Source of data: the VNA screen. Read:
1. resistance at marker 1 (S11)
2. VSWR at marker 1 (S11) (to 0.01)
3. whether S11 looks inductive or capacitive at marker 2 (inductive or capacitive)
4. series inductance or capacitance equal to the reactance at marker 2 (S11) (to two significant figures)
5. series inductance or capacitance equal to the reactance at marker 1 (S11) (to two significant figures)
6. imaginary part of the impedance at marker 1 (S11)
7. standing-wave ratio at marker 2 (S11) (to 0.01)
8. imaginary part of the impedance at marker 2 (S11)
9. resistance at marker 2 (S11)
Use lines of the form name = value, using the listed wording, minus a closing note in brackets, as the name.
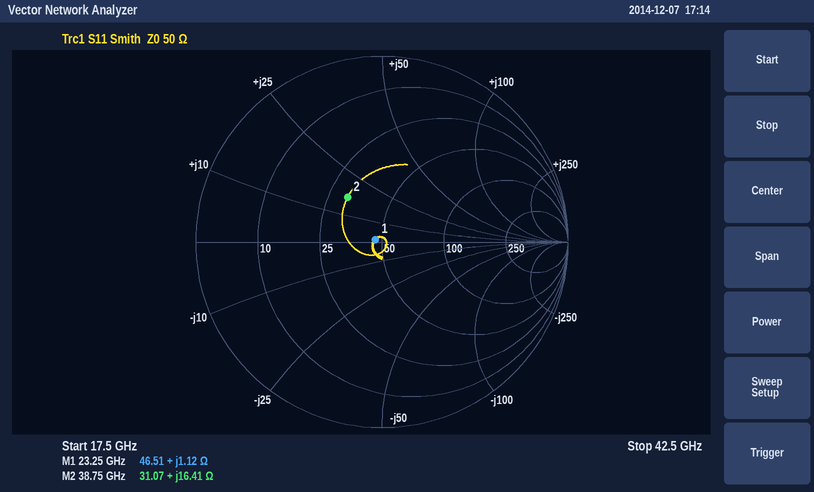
resistance at marker 1 = 46.51 Ω
VSWR at marker 1 (S11) = 1.08
whether S11 looks inductive or capacitive at marker 2 = inductive
series inductance or capacitance equal to the reactance at marker 2 (S11) = 67 pH
series inductance or capacitance equal to the reactance at marker 1 (S11) = 7.7 pH
imaginary part of the impedance at marker 1 = +1.12 Ω
standing-wave ratio at marker 2 (S11) = 1.87
imaginary part of the impedance at marker 2 = +16.41 Ω
resistance at marker 2 = 31.07 Ω
